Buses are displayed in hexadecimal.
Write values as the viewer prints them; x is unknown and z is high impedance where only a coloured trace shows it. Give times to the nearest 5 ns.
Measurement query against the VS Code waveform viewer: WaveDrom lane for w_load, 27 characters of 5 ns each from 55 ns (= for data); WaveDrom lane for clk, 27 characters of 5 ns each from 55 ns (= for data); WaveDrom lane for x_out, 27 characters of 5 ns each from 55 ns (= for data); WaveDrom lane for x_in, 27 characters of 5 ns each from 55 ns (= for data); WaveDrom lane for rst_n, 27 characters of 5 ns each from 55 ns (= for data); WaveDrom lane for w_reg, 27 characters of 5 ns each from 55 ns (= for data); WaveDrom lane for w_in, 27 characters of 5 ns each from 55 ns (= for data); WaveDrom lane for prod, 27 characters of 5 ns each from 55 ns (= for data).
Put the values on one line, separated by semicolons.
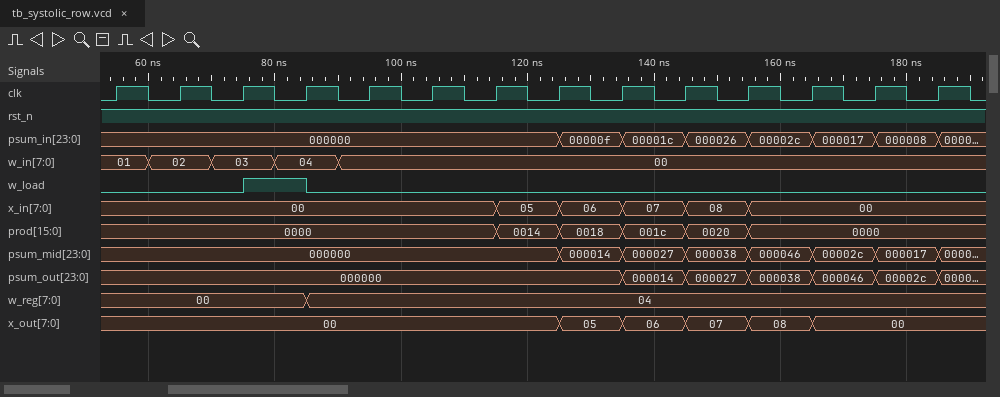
{name: 'w_load', wave: '0...1.0....................'}; {name: 'clk', wave: '101010101010101010101010101'}; {name: 'x_out', wave: '=.............=.=.=.=.=....', data: '00 05 06 07 08 00'}; {name: 'x_in', wave: '=...........=.=.=.=.=......', data: '00 05 06 07 08 00'}; {name: 'rst_n', wave: '1..........................'}; {name: 'w_reg', wave: '=.....=....................', data: '00 04'}; {name: 'w_in', wave: '==.=.=.=...................', data: '01 02 03 04 00'}; {name: 'prod', wave: '=...........=.=.=.=.=......', data: '0000 0014 0018 001c 0020 0000'}
